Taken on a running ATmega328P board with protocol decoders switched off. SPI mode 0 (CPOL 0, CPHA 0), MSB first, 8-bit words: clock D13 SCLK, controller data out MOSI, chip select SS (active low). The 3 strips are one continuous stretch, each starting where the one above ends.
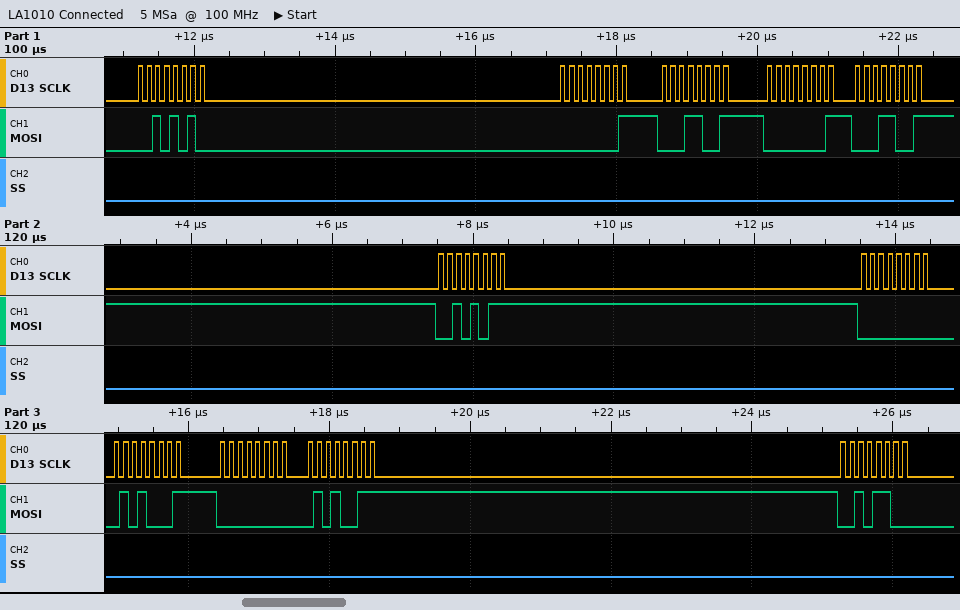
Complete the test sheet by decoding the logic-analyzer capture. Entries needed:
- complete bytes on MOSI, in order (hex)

2A 01 19 01 19 2B 00 51 00 53 2C
